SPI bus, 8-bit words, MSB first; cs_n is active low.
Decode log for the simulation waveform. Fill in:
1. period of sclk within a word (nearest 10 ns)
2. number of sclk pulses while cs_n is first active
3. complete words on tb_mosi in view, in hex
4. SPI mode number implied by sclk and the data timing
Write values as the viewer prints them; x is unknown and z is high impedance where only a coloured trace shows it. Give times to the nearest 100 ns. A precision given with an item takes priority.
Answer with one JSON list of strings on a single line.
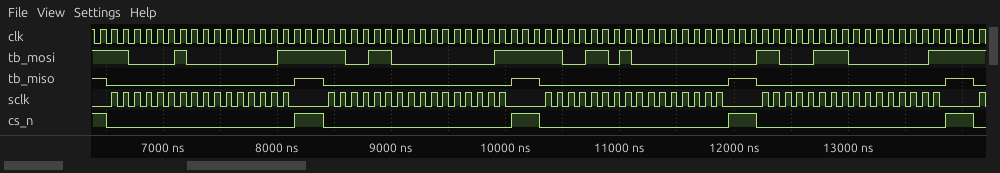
["100 ns", "16", "C2, 01, CC, 01, CD, 00, C7, 01", "0"]
